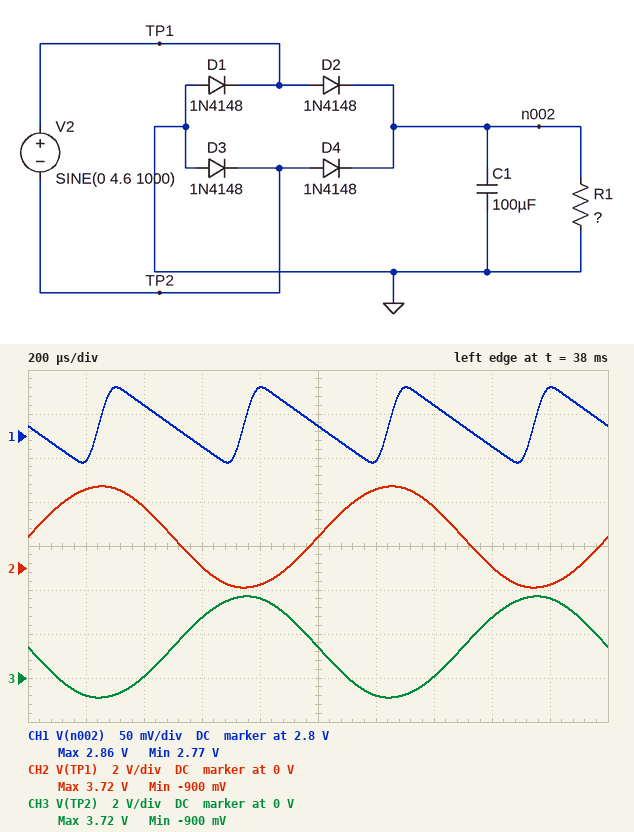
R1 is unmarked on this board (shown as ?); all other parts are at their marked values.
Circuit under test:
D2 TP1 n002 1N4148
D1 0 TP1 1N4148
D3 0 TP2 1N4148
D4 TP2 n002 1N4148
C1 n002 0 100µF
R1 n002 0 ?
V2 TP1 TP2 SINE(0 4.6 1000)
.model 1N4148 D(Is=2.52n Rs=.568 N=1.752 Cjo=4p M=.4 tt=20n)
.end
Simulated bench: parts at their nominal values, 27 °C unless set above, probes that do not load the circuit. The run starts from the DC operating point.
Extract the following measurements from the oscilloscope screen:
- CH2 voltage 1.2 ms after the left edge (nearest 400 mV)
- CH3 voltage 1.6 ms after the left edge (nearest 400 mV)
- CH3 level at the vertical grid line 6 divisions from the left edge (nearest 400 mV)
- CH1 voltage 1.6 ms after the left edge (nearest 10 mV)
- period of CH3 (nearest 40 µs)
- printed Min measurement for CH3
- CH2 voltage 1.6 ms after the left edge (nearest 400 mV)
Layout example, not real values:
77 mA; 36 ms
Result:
3.6 V; 2.8 V; -800 mV; 2.79 V; 1.00 ms; -900 mV; 0 V
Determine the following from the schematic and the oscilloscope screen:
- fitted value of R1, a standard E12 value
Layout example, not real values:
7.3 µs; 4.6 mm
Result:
120 Ω
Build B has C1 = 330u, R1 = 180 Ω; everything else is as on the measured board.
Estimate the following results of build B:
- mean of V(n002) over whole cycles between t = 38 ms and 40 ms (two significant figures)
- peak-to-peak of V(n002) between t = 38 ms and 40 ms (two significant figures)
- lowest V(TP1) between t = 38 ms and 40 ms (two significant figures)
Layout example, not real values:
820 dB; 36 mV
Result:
2.9 V; 18 mV; -860 mV
